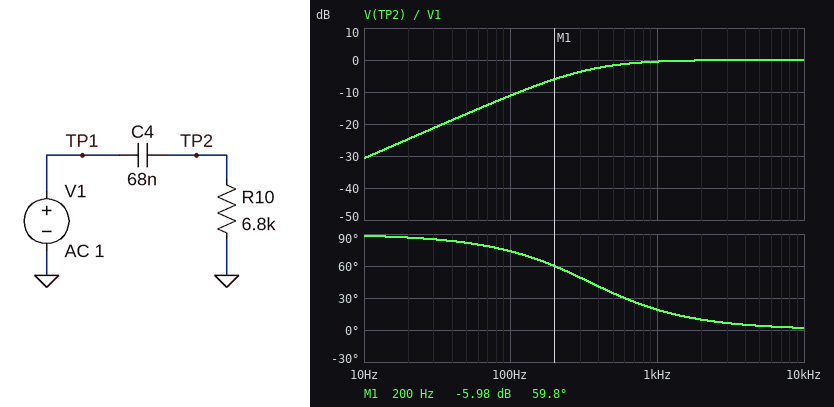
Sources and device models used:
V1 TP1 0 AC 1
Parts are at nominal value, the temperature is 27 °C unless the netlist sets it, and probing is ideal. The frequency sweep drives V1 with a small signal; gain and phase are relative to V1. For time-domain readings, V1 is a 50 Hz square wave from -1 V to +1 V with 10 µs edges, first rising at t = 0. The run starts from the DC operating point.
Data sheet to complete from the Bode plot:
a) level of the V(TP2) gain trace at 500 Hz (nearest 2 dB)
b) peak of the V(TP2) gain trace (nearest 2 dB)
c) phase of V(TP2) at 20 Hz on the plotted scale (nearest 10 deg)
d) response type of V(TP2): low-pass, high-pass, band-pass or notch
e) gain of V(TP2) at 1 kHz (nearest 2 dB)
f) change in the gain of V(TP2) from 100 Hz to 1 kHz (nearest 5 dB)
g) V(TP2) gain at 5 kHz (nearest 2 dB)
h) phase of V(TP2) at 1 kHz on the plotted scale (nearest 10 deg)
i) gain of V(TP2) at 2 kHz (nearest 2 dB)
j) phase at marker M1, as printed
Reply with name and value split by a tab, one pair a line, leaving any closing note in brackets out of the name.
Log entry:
level of the V(TP2) gain trace at 500 Hz	-2 dB
peak of the V(TP2) gain trace	0 dB
phase of V(TP2) at 20 Hz on the plotted scale	90 deg
response type of V(TP2): low-pass, high-pass, band-pass or notch	high-pass
gain of V(TP2) at 1 kHz	0 dB
change in the gain of V(TP2) from 100 Hz to 1 kHz	10 dB
V(TP2) gain at 5 kHz	0 dB
phase of V(TP2) at 1 kHz on the plotted scale	20 deg
gain of V(TP2) at 2 kHz	0 dB
phase at marker M1, as printed	59.8 deg
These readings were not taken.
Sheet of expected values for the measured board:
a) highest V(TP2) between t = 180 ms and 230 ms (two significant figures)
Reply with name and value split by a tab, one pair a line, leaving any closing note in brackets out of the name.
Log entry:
highest V(TP2) between t = 180 ms and 230 ms	2.0 V
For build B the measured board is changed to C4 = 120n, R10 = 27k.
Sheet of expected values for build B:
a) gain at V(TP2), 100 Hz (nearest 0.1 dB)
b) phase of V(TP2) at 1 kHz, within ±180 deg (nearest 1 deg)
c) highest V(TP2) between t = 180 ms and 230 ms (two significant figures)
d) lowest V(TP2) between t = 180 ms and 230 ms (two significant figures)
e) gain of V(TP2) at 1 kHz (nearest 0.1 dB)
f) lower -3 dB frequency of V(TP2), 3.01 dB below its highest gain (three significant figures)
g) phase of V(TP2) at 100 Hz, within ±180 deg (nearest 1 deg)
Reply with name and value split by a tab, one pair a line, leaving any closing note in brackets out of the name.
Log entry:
gain at V(TP2), 100 Hz	-0.9 dB
phase of V(TP2) at 1 kHz, within ±180 deg	3 deg
highest V(TP2) between t = 180 ms and 230 ms	1.9 V
lowest V(TP2) between t = 180 ms and 230 ms	-1.9 V
gain of V(TP2) at 1 kHz	0 dB
lower -3 dB frequency of V(TP2), 3.01 dB below its highest gain	49.1 Hz
phase of V(TP2) at 100 Hz, within ±180 deg	26 deg
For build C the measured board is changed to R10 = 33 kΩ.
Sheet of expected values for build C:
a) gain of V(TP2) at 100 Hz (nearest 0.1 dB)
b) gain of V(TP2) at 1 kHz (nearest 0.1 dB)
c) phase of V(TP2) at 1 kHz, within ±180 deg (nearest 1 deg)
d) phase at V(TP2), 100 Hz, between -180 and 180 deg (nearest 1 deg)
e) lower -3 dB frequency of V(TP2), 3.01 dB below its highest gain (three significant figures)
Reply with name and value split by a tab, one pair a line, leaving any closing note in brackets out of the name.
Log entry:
gain of V(TP2) at 100 Hz	-1.8 dB
gain of V(TP2) at 1 kHz	0 dB
phase of V(TP2) at 1 kHz, within ±180 deg	4 deg
phase at V(TP2), 100 Hz, between -180 and 180 deg	35 deg
lower -3 dB frequency of V(TP2), 3.01 dB below its highest gain	70.9 Hz
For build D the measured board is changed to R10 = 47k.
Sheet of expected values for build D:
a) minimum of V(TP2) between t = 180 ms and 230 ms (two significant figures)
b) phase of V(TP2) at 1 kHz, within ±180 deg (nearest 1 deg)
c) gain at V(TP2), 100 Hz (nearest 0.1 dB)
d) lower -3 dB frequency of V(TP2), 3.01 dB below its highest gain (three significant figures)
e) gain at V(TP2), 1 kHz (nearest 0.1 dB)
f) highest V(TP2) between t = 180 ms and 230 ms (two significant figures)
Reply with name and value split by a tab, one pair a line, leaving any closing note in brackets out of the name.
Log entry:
minimum of V(TP2) between t = 180 ms and 230 ms	-1.9 V
phase of V(TP2) at 1 kHz, within ±180 deg	3 deg
gain at V(TP2), 100 Hz	-1.0 dB
lower -3 dB frequency of V(TP2), 3.01 dB below its highest gain	49.8 Hz
gain at V(TP2), 1 kHz	0 dB
highest V(TP2) between t = 180 ms and 230 ms	1.9 V
